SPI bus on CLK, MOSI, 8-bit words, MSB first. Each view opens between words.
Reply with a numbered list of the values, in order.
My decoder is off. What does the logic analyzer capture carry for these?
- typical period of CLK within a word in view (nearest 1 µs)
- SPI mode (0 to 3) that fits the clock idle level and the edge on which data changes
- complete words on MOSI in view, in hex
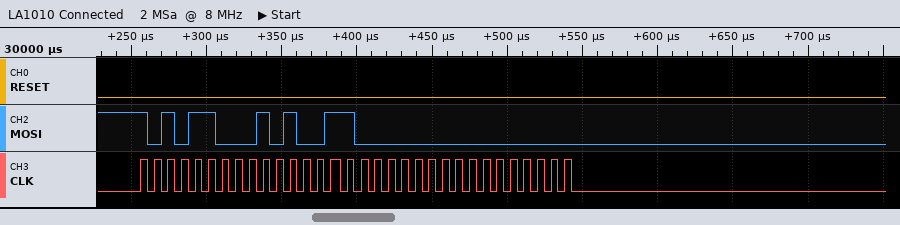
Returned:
1. 9 µs
2. 0
3. AC, 53, 00, 00
